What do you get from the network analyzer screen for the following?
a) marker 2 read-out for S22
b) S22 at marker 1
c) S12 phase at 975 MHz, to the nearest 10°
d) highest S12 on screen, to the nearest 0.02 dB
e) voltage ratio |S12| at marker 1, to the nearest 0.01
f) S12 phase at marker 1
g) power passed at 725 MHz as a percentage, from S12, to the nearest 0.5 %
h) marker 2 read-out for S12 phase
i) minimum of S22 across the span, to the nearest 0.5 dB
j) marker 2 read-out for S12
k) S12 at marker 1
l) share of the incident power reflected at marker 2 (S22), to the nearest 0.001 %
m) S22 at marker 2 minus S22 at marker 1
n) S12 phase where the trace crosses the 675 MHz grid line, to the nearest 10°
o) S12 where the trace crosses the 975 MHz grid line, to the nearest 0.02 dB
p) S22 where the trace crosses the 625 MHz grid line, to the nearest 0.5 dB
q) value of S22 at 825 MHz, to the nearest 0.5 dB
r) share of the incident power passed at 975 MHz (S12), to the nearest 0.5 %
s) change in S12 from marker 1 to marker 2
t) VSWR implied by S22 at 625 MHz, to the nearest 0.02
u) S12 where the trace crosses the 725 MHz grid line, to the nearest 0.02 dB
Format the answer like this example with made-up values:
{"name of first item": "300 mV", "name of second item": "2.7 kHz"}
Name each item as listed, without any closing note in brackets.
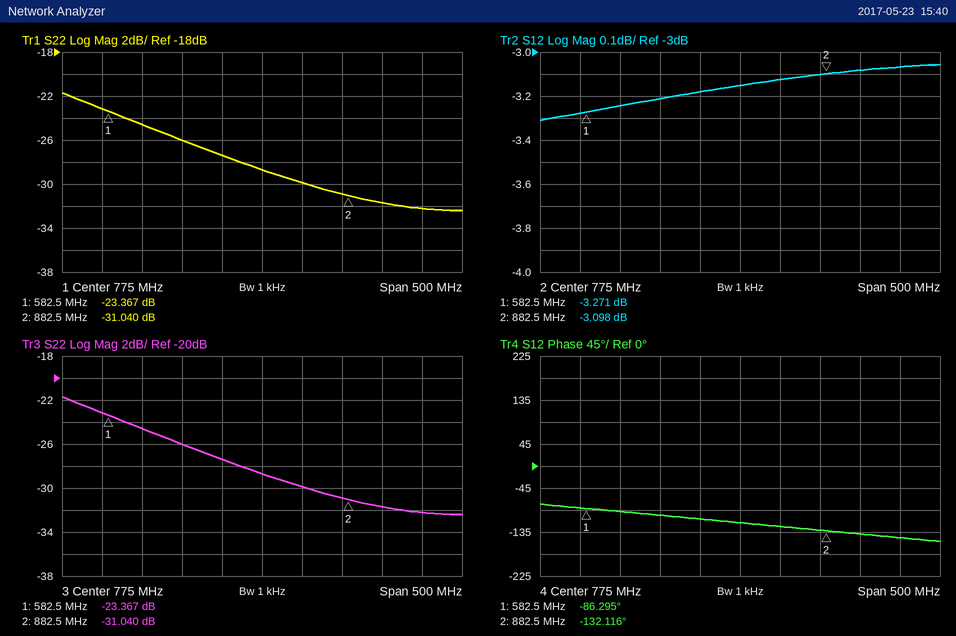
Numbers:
{"marker 2 read-out for S22": "-31.040 dB", "S22 at marker 1": "-23.367 dB", "S12 phase at 975 MHz, to the nearest 10°": "-150°", "highest S12 on screen, to the nearest 0.02 dB": "-3.06 dB", "voltage ratio |S12| at marker 1, to the nearest 0.01": "0.69", "S12 phase at marker 1": "-86.295°", "power passed at 725 MHz as a percentage, from S12, to the nearest 0.5 %": "48.0 %", "marker 2 read-out for S12 phase": "-132.116°", "minimum of S22 across the span, to the nearest 0.5 dB": "-32.5 dB", "marker 2 read-out for S12": "-3.098 dB", "S12 at marker 1": "-3.271 dB", "share of the incident power reflected at marker 2 (S22), to the nearest 0.001 %": "0.079 %", "S22 at marker 2 minus S22 at marker 1": "-7.673 dB", "S12 phase where the trace crosses the 675 MHz grid line, to the nearest 10°": "-100°", "S12 where the trace crosses the 975 MHz grid line, to the nearest 0.02 dB": "-3.06 dB", "S22 where the trace crosses the 625 MHz grid line, to the nearest 0.5 dB": "-24.5 dB", "value of S22 at 825 MHz, to the nearest 0.5 dB": "-30.0 dB", "share of the incident power passed at 975 MHz (S12), to the nearest 0.5 %": "49.5 %", "change in S12 from marker 1 to marker 2": "0.173 dB", "VSWR implied by S22 at 625 MHz, to the nearest 0.02": "1.12", "S12 where the trace crosses the 725 MHz grid line, to the nearest 0.02 dB": "-3.18 dB"}
